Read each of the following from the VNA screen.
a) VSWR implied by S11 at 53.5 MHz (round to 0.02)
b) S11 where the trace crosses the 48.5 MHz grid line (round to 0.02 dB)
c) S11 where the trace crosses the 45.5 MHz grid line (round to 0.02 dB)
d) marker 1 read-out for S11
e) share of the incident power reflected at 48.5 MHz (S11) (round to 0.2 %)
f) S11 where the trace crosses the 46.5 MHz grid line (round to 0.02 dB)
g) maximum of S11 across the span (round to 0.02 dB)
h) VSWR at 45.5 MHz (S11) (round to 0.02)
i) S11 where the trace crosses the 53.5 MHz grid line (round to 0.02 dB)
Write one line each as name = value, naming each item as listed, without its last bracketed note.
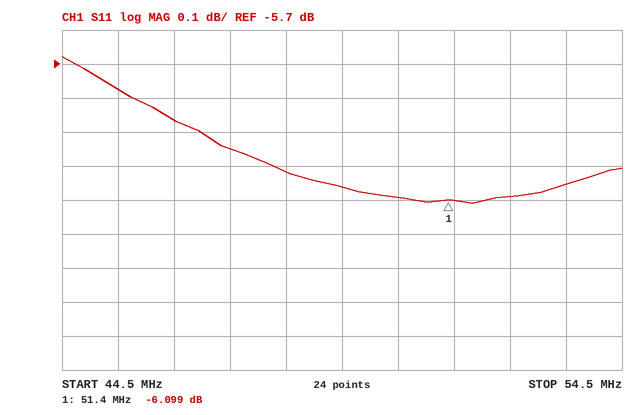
VSWR implied by S11 at 53.5 MHz = 2.98
S11 where the trace crosses the 48.5 MHz grid line = -6.02 dB
S11 where the trace crosses the 45.5 MHz grid line = -5.78 dB
marker 1 read-out for S11 = -6.099 dB
share of the incident power reflected at 48.5 MHz (S11) = 25.0 %
S11 where the trace crosses the 46.5 MHz grid line = -5.86 dB
maximum of S11 across the span = -5.68 dB
VSWR at 45.5 MHz (S11) = 3.12
S11 where the trace crosses the 53.5 MHz grid line = -6.06 dB
